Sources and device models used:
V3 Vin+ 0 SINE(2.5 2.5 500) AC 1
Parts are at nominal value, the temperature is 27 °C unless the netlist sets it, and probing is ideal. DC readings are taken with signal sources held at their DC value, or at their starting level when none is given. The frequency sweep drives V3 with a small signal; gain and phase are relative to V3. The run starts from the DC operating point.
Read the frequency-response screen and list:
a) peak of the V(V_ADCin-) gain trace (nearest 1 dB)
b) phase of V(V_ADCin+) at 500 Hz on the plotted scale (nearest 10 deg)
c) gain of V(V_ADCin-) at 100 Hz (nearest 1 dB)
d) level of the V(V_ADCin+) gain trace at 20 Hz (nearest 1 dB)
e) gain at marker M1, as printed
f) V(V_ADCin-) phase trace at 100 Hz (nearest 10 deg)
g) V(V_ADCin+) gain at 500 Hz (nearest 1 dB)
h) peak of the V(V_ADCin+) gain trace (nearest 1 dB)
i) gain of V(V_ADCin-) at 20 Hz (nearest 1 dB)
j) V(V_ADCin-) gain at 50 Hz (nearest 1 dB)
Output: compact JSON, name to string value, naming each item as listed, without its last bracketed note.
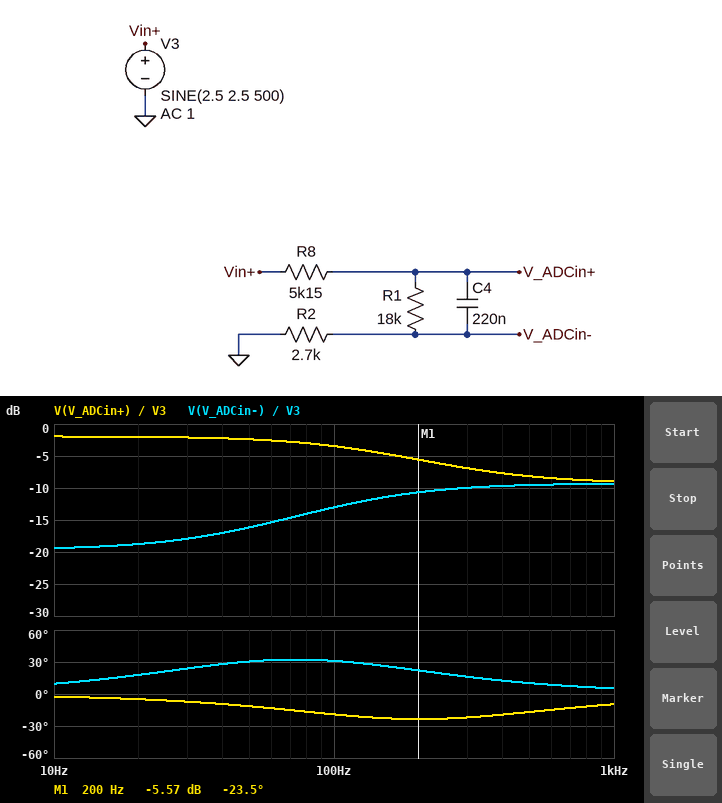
{"peak of the V(V_ADCin-) gain trace": "-9 dB", "phase of V(V_ADCin+) at 500 Hz on the plotted scale": "-20 deg", "gain of V(V_ADCin-) at 100 Hz": "-13 dB", "level of the V(V_ADCin+) gain trace at 20 Hz": "-2 dB", "gain at marker M1, as printed": "-5.57 dB", "V(V_ADCin-) phase trace at 100 Hz": "30 deg", "V(V_ADCin+) gain at 500 Hz": "-8 dB", "peak of the V(V_ADCin+) gain trace": "-2 dB", "gain of V(V_ADCin-) at 20 Hz": "-19 dB", "V(V_ADCin-) gain at 50 Hz": "-16 dB"}
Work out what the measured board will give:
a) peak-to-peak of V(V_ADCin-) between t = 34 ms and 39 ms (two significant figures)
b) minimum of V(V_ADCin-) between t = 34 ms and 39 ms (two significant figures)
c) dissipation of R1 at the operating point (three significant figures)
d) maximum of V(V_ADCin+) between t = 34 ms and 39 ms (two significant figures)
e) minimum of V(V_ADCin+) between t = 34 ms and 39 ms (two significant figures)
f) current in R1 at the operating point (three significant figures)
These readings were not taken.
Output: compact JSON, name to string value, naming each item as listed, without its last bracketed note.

{"peak-to-peak of V(V_ADCin-) between t = 34 ms and 39 ms": "1.7 V", "minimum of V(V_ADCin-) between t = 34 ms and 39 ms": "-570 mV", "dissipation of R1 at the operating point": "168 µW", "maximum of V(V_ADCin+) between t = 34 ms and 39 ms": "3.0 V", "minimum of V(V_ADCin+) between t = 34 ms and 39 ms": "1.0 V", "current in R1 at the operating point": "96.7 µA"}
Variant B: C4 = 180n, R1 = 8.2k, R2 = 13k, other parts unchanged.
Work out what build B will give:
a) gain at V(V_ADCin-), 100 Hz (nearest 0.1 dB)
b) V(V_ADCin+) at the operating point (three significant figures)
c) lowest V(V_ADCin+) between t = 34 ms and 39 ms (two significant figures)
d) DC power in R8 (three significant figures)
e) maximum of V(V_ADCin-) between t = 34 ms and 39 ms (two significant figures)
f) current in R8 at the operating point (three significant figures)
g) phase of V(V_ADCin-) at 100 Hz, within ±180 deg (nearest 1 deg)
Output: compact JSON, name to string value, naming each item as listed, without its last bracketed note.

{"gain at V(V_ADCin-), 100 Hz": "-4.9 dB", "V(V_ADCin+) at the operating point": "2.01 V", "lowest V(V_ADCin+) between t = 34 ms and 39 ms": "200 mV", "DC power in R8": "46.4 µW", "maximum of V(V_ADCin-) between t = 34 ms and 39 ms": "3.0 V", "current in R8 at the operating point": "94.9 µA", "phase of V(V_ADCin-) at 100 Hz, within ±180 deg": "10 deg"}
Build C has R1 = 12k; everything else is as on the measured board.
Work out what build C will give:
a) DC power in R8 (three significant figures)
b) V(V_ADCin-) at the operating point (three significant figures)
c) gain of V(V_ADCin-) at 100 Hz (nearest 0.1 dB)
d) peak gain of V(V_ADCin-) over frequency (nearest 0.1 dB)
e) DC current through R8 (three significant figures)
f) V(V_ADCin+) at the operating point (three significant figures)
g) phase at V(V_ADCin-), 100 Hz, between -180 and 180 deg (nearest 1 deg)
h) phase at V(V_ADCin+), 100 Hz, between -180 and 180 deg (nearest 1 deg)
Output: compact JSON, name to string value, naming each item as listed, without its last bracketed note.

{"DC power in R8": "81.7 µW", "V(V_ADCin-) at the operating point": "340 mV", "gain of V(V_ADCin-) at 100 Hz": "-13.1 dB", "peak gain of V(V_ADCin-) over frequency": "-9.3 dB", "DC current through R8": "126 µA", "V(V_ADCin+) at the operating point": "1.85 V", "phase at V(V_ADCin-), 100 Hz, between -180 and 180 deg": "26 deg", "phase at V(V_ADCin+), 100 Hz, between -180 and 180 deg": "-16 deg"}
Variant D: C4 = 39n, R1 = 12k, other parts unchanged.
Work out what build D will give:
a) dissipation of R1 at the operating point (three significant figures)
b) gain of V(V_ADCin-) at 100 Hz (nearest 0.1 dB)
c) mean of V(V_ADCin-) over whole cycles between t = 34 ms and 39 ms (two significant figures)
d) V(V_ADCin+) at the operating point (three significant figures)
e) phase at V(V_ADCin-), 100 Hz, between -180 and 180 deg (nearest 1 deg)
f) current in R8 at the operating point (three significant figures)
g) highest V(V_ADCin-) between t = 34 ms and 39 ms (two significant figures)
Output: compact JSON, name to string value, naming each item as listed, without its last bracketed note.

{"dissipation of R1 at the operating point": "190 µW", "gain of V(V_ADCin-) at 100 Hz": "-17.0 dB", "mean of V(V_ADCin-) over whole cycles between t = 34 ms and 39 ms": "340 mV", "V(V_ADCin+) at the operating point": "1.85 V", "phase at V(V_ADCin-), 100 Hz, between -180 and 180 deg": "10 deg", "current in R8 at the operating point": "126 µA", "highest V(V_ADCin-) between t = 34 ms and 39 ms": "860 mV"}
